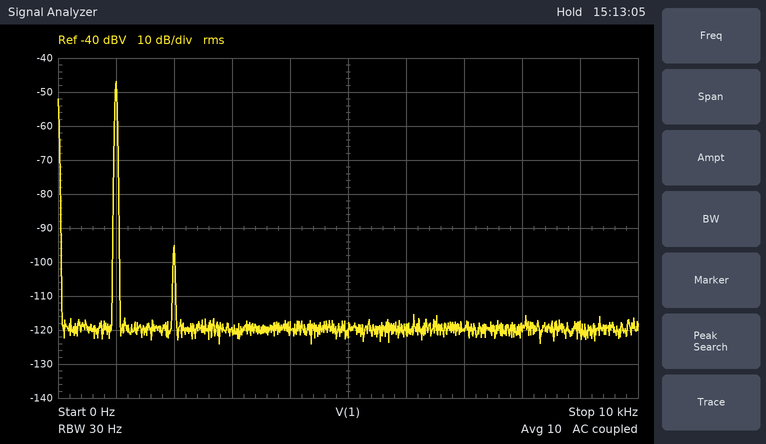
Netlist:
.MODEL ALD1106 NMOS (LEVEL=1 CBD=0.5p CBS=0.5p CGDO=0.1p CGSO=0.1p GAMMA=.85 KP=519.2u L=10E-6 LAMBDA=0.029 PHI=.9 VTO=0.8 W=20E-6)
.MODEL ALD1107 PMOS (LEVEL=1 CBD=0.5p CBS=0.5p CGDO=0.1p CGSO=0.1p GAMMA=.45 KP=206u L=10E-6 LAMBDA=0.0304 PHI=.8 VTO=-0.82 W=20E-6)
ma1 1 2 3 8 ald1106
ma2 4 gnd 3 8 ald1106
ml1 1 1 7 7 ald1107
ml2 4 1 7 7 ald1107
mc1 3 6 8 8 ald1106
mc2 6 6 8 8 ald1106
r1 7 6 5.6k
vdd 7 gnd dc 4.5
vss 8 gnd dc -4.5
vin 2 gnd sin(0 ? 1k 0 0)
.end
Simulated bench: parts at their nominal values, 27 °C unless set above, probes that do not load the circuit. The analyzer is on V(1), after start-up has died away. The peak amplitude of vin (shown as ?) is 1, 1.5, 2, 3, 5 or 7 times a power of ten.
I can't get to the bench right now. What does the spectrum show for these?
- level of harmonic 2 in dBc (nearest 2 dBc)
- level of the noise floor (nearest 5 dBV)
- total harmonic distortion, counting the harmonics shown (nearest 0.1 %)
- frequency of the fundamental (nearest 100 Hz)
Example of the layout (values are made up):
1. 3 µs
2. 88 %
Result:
1. -48 dBc
2. -120 dBV
3. 0.4 %
4. 1.0 kHz
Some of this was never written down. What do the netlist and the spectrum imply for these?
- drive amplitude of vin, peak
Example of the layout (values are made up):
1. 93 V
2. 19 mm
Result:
1. 15 mV
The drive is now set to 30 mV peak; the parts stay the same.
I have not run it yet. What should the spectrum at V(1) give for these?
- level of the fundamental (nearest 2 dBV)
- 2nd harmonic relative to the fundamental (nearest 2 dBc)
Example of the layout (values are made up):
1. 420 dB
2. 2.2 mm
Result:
1. -40 dBV
2. -30 dBc
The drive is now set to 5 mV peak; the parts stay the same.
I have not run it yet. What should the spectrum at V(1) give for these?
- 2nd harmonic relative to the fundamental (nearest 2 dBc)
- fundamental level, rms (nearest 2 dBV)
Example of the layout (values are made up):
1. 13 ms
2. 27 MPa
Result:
1. -58 dBc
2. -56 dBV
